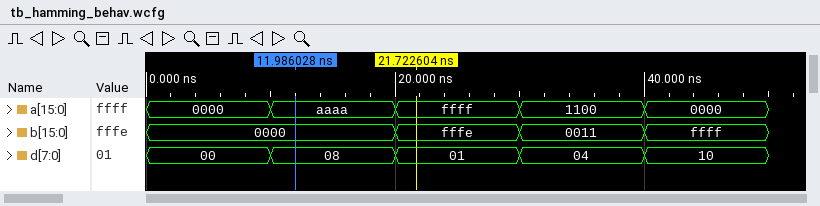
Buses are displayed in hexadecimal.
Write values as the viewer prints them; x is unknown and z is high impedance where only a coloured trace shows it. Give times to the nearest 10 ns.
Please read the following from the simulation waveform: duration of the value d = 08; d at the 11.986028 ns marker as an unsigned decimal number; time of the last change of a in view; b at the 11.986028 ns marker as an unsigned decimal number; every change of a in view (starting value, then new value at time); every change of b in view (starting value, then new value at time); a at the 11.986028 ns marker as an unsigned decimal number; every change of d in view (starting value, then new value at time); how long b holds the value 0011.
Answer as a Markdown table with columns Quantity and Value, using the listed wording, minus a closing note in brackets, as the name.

| Quantity | Value |
|---|---|
| duration of the value d = 08 | 10 ns |
| d at the 11.986028 ns marker as an unsigned decimal number | 8 |
| time of the last change of a in view | 40 ns |
| b at the 11.986028 ns marker as an unsigned decimal number | 0 |
| every change of a in view | 0000, aaaa at 10 ns, ffff at 20 ns, 1100 at 30 ns, 0000 at 40 ns |
| every change of b in view | 0000, fffe at 20 ns, 0011 at 30 ns, ffff at 40 ns |
| a at the 11.986028 ns marker as an unsigned decimal number | 43690 |
| every change of d in view | 00, 08 at 10 ns, 01 at 20 ns, 04 at 30 ns, 10 at 40 ns |
| how long b holds the value 0011 | 10 ns |
